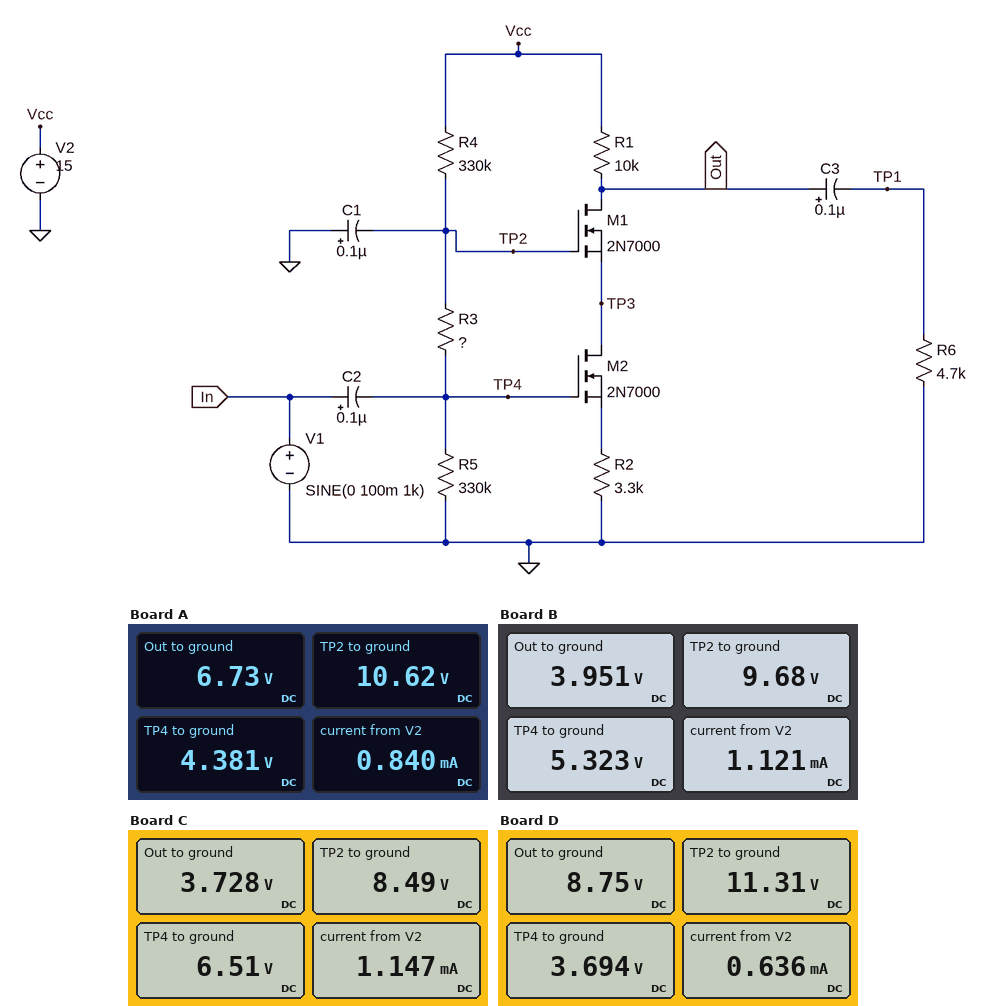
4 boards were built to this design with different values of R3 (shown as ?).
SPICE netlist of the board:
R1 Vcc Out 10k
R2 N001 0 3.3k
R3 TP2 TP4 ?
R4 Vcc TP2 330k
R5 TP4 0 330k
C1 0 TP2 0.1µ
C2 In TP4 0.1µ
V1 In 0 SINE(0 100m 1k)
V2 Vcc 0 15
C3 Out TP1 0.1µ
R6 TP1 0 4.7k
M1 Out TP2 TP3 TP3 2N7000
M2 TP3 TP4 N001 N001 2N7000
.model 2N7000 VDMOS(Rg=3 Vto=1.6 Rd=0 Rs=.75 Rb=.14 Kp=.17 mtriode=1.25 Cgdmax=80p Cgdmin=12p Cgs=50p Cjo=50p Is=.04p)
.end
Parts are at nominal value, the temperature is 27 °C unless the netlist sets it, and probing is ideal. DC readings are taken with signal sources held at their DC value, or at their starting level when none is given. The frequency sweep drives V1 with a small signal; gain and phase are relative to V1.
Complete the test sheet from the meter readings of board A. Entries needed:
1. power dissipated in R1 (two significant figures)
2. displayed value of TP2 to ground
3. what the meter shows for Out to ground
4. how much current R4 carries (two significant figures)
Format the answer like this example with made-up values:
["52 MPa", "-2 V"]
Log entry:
["6.8 mW", "10.62 V", "6.73 V", "13 µA"]
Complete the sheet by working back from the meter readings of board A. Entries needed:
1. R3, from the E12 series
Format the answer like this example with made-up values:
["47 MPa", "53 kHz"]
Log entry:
["470 kΩ"]
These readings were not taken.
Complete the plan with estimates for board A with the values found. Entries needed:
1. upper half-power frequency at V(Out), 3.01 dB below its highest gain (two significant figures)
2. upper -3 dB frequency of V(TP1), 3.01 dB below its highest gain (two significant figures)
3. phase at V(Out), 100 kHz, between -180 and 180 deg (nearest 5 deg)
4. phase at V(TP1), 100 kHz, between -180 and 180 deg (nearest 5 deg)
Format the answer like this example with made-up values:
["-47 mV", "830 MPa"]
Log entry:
["140 Hz", "340 kHz", "160 deg", "160 deg"]
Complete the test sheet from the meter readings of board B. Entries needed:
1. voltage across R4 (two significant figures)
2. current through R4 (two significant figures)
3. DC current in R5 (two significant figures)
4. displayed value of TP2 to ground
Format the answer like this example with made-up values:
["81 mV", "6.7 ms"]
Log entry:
["5.3 V", "16 µA", "16 µA", "9.68 V"]
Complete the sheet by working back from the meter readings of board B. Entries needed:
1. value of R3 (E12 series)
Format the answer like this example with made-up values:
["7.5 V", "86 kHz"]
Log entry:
["270 kΩ"]
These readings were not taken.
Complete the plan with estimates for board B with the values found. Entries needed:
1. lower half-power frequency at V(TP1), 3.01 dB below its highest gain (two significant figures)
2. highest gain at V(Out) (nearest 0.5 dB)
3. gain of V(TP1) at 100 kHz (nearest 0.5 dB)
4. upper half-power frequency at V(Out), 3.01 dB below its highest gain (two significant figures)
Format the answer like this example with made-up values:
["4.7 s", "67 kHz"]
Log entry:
["110 Hz", "8.5 dB", "-1.0 dB", "150 Hz"]
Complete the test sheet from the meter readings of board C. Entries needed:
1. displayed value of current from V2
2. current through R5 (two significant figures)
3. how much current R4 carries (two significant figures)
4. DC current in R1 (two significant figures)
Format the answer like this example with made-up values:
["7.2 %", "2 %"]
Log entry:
["1.147 mA", "20 µA", "20 µA", "1.1 mA"]
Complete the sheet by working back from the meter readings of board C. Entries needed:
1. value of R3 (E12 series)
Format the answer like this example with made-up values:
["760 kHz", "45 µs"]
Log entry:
["100 kΩ"]
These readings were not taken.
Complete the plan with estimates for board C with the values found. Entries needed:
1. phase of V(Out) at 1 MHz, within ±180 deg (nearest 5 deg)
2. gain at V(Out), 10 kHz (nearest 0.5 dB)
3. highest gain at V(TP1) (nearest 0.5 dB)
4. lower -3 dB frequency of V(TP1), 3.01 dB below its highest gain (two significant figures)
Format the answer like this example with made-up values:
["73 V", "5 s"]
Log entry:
["20 deg", "-37.5 dB", "-6.0 dB", "380 kHz"]
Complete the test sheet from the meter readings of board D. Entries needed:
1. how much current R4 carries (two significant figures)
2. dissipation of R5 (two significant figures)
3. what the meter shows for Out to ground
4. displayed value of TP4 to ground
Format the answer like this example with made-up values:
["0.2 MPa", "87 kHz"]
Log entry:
["11 µA", "41 µW", "8.75 V", "3.694 V"]
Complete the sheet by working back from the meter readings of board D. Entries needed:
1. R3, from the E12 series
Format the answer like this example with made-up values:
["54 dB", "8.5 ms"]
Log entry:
["680 kΩ"]
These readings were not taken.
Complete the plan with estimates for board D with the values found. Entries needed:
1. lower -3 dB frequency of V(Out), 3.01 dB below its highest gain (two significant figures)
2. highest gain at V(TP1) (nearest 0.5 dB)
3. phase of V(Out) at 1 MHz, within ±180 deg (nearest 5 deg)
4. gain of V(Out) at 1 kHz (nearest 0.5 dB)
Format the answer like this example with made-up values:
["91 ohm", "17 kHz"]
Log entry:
["6.3 Hz", "-0.5 dB", "85 deg", "0 dB"]
